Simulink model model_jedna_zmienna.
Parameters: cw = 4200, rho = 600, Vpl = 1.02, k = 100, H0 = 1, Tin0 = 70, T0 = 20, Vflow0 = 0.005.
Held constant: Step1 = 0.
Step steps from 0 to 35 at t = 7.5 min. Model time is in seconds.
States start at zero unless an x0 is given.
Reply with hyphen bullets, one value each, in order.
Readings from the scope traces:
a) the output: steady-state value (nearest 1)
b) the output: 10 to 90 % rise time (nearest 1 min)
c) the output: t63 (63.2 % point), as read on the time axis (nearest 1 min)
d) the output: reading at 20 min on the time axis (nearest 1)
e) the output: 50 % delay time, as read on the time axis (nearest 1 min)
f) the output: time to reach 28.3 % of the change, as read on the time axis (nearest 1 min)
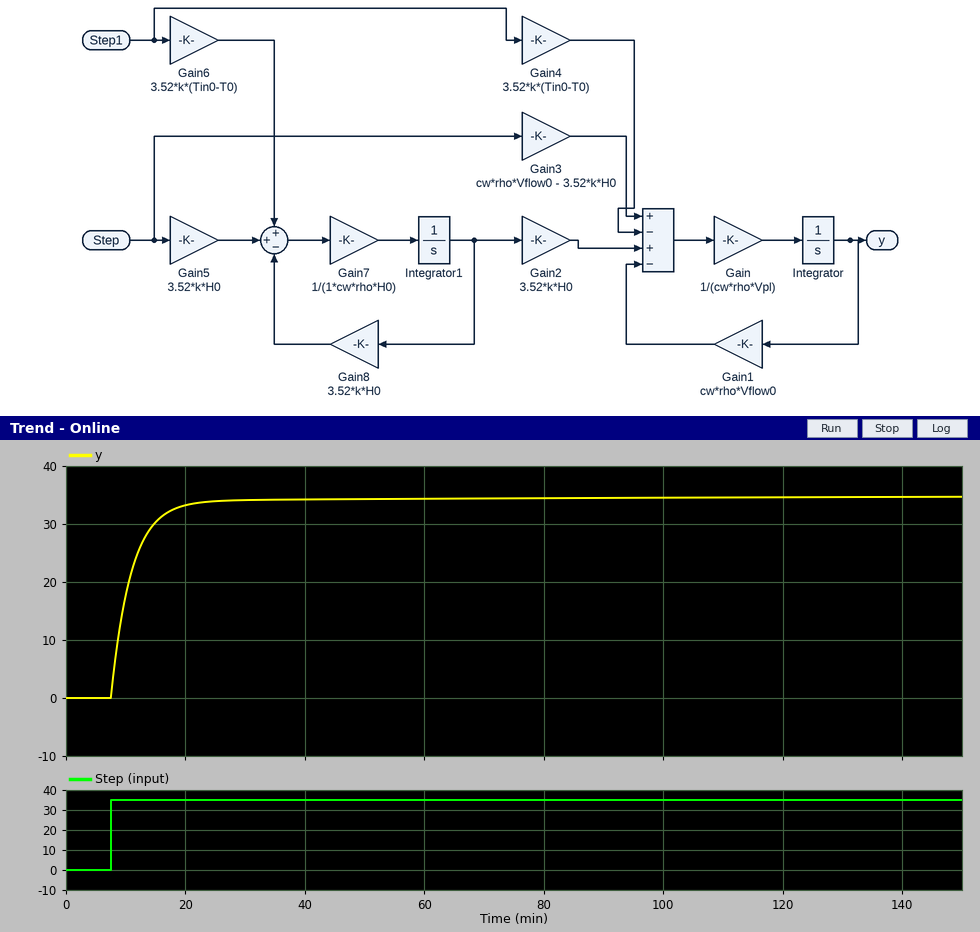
- 35
- 8 min
- 11 min
- 33
- 10 min
- 9 min
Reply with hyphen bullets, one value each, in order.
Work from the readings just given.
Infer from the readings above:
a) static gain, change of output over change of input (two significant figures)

- 1.0
